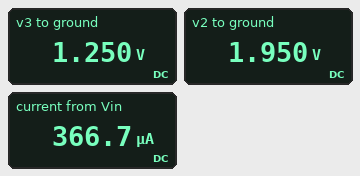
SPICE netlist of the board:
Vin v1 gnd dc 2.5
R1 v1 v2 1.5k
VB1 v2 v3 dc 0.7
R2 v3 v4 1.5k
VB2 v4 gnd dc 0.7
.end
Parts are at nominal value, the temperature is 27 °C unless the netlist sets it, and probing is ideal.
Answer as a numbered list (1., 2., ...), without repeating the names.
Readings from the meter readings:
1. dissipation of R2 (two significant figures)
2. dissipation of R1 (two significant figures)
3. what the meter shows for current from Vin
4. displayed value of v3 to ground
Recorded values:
1. 200 µW
2. 200 µW
3. 366.7 µA
4. 1.250 V
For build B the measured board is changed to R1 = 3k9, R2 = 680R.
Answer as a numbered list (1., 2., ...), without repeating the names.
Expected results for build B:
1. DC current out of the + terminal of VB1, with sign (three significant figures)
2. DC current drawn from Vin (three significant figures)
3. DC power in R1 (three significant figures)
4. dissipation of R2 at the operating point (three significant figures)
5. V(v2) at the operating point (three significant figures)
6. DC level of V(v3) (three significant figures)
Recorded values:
1. -240 µA
2. 240 µA
3. 225 µW
4. 39.2 µW
5. 1.56 V
6. 863 mV
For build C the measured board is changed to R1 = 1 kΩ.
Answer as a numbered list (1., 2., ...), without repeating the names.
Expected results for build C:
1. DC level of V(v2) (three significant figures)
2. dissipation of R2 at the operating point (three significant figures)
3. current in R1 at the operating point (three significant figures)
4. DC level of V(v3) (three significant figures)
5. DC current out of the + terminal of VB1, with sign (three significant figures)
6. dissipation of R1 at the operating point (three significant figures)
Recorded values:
1. 2.06 V
2. 290 µW
3. 440 µA
4. 1.36 V
5. -440 µA
6. 194 µW
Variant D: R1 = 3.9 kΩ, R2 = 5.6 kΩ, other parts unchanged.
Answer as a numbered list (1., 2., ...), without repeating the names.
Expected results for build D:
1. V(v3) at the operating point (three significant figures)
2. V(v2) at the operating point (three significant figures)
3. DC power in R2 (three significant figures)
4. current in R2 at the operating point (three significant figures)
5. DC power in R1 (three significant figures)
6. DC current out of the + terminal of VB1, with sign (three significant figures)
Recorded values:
1. 1.35 V
2. 2.05 V
3. 75.1 µW
4. 116 µA
5. 52.3 µW
6. -116 µA
